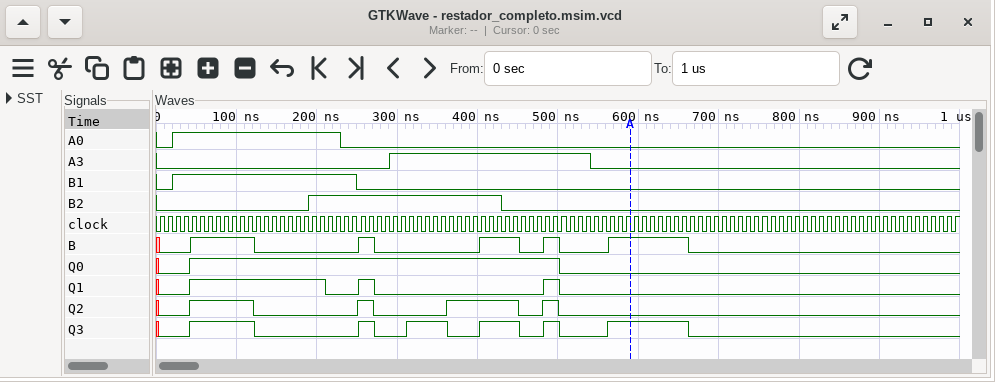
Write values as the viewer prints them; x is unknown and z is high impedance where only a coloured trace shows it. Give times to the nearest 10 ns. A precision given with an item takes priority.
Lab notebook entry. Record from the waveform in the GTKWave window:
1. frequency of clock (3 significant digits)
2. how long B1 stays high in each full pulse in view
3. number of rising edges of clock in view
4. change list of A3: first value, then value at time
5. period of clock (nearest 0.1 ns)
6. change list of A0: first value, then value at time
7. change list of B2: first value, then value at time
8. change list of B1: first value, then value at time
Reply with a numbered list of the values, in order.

1. 100 MHz
2. 230 ns
3. 100
4. 0, 1 at 290 ns, 0 at 540 ns
5. 10 ns
6. 0, 1 at 20 ns, 0 at 230 ns
7. 0, 1 at 190 ns, 0 at 430 ns
8. 0, 1 at 20 ns, 0 at 250 ns
